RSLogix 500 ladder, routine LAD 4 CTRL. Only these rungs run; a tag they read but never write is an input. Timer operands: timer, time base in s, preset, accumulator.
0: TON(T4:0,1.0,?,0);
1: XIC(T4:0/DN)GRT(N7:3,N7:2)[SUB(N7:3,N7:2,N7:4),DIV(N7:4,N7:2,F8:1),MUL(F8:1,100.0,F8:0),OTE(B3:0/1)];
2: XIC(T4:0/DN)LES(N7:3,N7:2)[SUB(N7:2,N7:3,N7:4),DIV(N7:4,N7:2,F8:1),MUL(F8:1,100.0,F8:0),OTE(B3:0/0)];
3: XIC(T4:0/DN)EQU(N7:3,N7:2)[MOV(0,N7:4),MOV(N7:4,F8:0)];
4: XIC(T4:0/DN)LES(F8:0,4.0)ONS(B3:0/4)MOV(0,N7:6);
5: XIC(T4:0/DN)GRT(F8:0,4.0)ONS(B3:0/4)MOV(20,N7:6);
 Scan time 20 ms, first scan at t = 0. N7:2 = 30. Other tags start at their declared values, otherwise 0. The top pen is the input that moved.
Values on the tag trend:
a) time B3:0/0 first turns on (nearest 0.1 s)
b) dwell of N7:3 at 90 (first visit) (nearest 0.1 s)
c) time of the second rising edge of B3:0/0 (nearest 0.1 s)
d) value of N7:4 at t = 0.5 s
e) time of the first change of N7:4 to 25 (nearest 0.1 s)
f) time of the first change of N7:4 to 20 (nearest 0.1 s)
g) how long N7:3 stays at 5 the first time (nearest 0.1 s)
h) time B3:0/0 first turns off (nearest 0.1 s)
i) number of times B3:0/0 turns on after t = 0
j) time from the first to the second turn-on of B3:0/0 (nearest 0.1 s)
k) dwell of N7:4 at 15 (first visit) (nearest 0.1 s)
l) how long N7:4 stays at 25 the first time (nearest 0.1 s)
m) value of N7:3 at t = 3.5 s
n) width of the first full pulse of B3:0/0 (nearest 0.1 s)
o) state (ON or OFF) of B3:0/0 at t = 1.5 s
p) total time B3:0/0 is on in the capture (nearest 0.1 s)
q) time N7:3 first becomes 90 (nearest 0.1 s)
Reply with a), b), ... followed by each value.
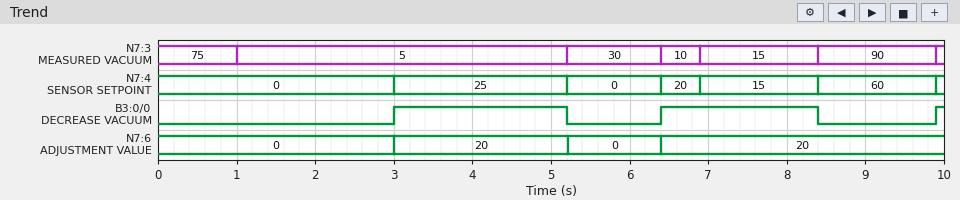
a) 3.0 s
b) 1.5 s
c) 6.4 s
d) 0
e) 3.0 s
f) 6.4 s
g) 4.2 s
h) 5.2 s
i) 3
j) 3.4 s
k) 1.5 s
l) 2.2 s
m) 5
n) 2.2 s
o) OFF
p) 4.3 s
q) 8.4 s
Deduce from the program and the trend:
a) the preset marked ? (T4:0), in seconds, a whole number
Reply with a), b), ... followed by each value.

a) 3 s
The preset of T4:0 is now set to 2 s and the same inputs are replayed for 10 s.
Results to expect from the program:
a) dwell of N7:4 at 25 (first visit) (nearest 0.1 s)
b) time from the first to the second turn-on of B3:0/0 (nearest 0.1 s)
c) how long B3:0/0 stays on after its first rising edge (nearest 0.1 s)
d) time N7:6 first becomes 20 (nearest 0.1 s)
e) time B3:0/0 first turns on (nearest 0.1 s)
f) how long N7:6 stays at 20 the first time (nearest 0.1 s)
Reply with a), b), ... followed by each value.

a) 3.2 s
b) 4.4 s
c) 3.2 s
d) 2.0 s
e) 2.0 s
f) 3.2 s
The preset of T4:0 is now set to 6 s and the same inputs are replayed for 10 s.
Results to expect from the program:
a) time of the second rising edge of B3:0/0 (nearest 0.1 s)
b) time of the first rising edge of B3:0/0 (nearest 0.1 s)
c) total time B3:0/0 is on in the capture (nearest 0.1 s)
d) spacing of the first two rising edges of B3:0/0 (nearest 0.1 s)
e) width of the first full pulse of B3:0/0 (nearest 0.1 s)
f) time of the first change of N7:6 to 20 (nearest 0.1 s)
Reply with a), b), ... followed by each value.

a) 9.9 s
b) 6.4 s
c) 2.1 s
d) 3.5 s
e) 2.0 s
f) 6.4 s
